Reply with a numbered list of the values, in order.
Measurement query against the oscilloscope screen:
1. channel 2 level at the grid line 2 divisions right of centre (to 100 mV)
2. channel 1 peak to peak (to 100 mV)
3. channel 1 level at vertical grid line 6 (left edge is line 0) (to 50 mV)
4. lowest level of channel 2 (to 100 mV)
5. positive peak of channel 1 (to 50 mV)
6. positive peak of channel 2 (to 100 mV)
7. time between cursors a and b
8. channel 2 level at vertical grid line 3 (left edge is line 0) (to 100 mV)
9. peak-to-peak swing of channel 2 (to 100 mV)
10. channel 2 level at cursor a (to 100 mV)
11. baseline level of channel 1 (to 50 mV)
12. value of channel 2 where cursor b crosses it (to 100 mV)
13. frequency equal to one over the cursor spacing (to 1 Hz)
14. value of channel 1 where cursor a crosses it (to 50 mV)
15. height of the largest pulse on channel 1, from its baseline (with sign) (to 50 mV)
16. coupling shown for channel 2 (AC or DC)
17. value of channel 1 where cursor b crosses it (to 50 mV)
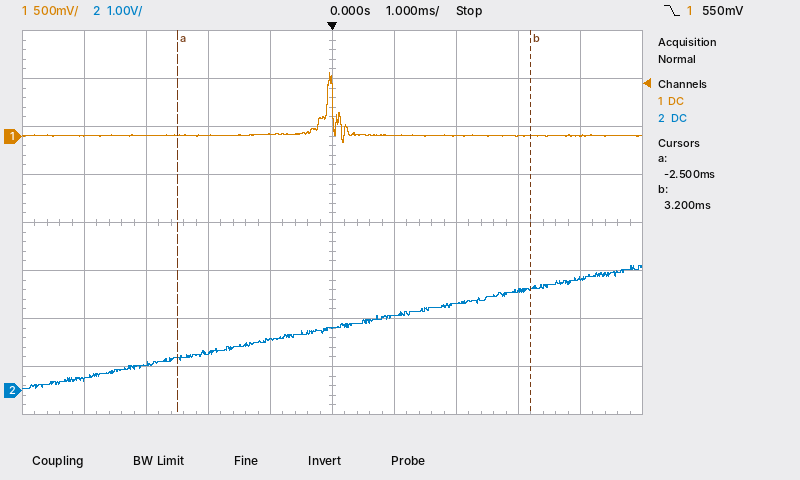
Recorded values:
1. 1.8 V
2. 700 mV
3. 0 mV
4. 0.0 V
5. 650 mV
6. 2.6 V
7. 5.7 ms
8. 800 mV
9. 2.6 V
10. 700 mV
11. 0 mV
12. 2.1 V
13. 175 Hz
14. 0 mV
15. +650 mV
16. DC
17. 0 mV
